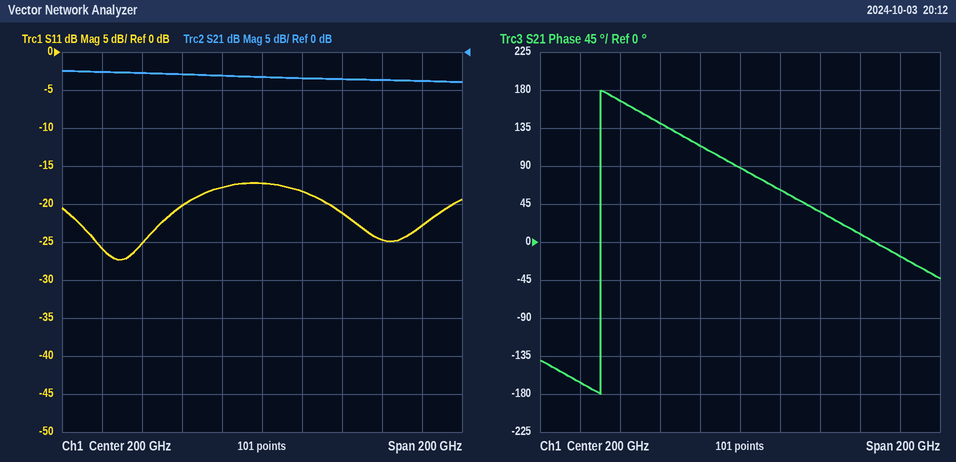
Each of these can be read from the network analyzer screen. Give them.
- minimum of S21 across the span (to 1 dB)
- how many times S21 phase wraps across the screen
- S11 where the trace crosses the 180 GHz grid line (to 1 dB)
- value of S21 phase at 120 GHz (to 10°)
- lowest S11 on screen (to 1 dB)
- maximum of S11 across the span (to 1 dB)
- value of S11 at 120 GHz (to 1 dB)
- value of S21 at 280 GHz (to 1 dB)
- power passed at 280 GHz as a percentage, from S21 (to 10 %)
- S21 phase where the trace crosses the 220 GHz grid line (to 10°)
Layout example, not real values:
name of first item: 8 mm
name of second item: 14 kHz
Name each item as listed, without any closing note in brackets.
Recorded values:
minimum of S21 across the span: -4 dB
how many times S21 phase wraps across the screen: 1
S11 where the trace crosses the 180 GHz grid line: -18 dB
value of S21 phase at 120 GHz: -170°
lowest S11 on screen: -27 dB
maximum of S11 across the span: -17 dB
value of S11 at 120 GHz: -26 dB
value of S21 at 280 GHz: -4 dB
power passed at 280 GHz as a percentage, from S21: 40 %
S21 phase where the trace crosses the 220 GHz grid line: 60°
